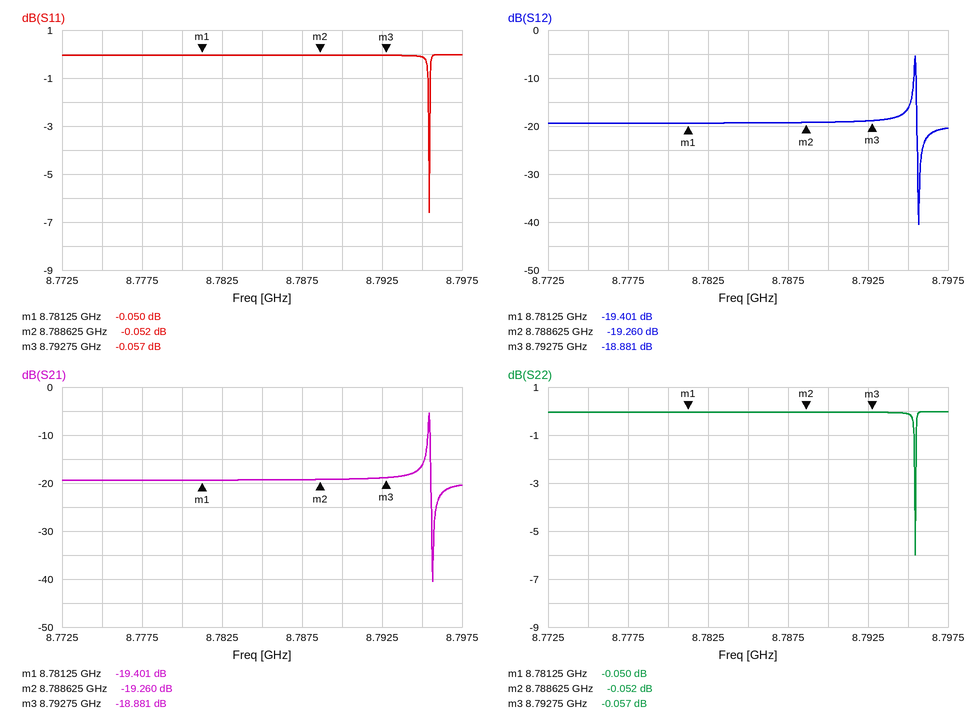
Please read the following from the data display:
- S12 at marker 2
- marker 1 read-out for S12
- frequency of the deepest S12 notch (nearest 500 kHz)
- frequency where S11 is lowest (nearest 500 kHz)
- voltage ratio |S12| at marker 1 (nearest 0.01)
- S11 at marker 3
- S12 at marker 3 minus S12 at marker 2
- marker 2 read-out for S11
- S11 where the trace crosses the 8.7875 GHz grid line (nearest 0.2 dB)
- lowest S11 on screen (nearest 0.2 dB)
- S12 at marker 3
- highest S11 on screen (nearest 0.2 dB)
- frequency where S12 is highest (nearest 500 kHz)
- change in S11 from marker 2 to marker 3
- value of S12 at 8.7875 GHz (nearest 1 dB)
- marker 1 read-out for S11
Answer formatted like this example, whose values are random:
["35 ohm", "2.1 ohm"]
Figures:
["-19.260 dB", "-19.401 dB", "8.7955 GHz", "8.7955 GHz", "0.11", "-0.057 dB", "0.379 dB", "-0.052 dB", "0.0 dB", "-6.6 dB", "-18.881 dB", "0.0 dB", "8.7955 GHz", "-0.005 dB", "-19 dB", "-0.050 dB"]
